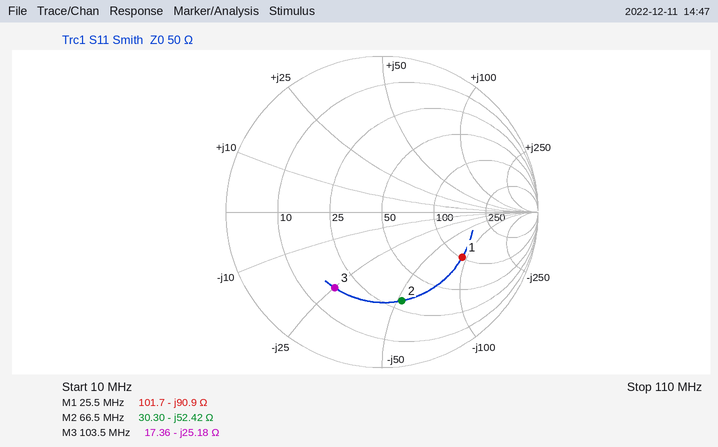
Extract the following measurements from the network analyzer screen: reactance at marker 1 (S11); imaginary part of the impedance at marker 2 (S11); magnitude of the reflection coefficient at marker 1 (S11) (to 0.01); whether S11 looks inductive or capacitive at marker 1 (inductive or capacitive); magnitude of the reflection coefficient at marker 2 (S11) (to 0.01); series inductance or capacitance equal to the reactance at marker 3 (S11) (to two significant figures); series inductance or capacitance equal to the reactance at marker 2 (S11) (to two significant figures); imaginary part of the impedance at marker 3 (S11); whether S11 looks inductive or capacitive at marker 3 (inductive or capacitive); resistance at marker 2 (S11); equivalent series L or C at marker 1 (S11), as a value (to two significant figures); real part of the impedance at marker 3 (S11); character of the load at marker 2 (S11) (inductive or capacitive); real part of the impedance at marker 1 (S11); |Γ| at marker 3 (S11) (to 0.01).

-90.9 Ω
-52.42 Ω
0.59
capacitive
0.58
61 pF
46 pF
-25.18 Ω
capacitive
30.30 Ω
69 pF
17.36 Ω
capacitive
101.7 Ω
0.57
